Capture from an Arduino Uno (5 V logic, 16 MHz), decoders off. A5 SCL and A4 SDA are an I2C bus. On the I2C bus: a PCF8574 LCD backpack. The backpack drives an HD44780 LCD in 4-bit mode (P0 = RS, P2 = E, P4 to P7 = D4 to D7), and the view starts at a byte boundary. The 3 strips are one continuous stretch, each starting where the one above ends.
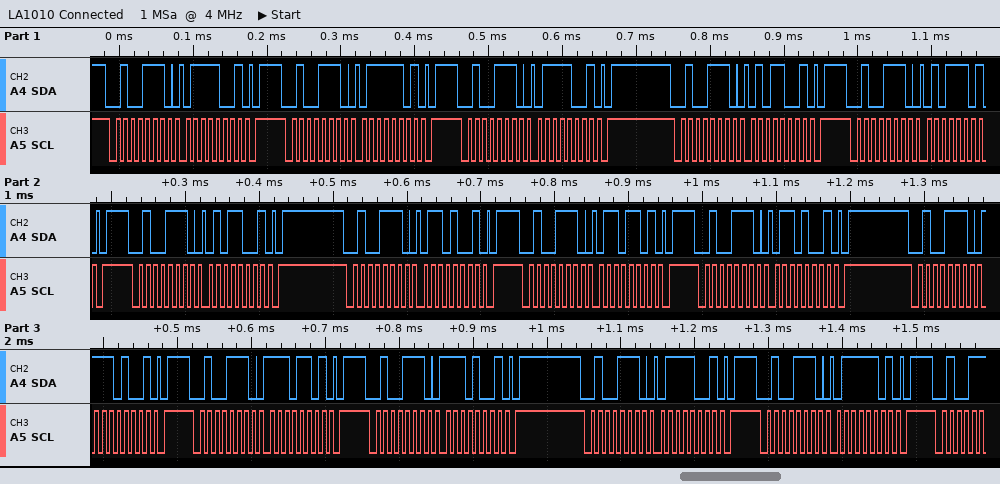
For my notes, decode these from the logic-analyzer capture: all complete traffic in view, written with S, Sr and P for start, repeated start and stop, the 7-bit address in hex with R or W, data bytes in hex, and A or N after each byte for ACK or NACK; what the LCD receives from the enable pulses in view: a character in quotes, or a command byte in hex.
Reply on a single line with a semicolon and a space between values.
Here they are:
S 27W A 79 A P S 27W A 7D A P S 27W A 79 A P S 27W A 59 A P S 27W A 5D A P S 27W A 59 A P S 27W A 69 A P S 27W A 6D A P S 27W A 69 A P S 27W A E9 A P S 27W A ED A P S 27W A E9 A P S 27W A 79 A P S 27W A 7D A P; 'u' 'n'
